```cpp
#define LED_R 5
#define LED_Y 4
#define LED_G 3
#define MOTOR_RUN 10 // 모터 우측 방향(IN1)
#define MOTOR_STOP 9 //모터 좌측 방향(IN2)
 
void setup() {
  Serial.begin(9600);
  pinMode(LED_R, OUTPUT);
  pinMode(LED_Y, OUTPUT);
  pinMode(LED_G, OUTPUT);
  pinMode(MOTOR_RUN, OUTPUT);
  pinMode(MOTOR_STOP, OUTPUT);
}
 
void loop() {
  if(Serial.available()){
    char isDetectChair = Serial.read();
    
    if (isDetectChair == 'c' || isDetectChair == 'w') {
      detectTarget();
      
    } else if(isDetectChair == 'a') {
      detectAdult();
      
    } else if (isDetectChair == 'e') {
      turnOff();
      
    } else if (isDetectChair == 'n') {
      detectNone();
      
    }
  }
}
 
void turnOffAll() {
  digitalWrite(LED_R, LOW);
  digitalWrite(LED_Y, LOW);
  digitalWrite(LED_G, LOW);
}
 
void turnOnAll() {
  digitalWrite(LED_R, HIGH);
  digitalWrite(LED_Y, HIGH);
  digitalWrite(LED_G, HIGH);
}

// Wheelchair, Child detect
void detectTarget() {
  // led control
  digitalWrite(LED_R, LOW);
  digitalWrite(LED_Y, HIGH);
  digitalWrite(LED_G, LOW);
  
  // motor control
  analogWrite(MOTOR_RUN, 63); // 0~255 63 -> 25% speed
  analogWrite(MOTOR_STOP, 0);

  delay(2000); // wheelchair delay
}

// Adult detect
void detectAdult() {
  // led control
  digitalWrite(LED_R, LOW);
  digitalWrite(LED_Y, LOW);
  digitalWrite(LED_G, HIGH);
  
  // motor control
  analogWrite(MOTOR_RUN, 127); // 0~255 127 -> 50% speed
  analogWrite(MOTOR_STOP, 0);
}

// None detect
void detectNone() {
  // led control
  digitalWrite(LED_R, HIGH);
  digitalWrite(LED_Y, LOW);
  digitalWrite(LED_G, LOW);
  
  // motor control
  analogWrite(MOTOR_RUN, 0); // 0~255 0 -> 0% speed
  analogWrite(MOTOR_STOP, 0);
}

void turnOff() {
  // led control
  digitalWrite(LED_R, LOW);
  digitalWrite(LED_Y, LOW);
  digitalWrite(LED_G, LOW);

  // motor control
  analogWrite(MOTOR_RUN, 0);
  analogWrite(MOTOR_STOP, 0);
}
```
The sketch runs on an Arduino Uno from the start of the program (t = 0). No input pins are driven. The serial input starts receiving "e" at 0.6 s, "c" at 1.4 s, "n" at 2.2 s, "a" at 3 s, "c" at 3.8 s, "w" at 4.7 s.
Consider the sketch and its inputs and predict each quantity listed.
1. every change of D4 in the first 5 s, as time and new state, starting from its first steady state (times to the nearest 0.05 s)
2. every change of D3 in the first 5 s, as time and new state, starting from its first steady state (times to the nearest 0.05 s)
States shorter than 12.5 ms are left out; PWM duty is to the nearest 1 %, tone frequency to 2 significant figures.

0 s low; 1.4 s high; 3.4 s low; 3.8 s high
0 s low; 3.4 s high; 3.8 s low
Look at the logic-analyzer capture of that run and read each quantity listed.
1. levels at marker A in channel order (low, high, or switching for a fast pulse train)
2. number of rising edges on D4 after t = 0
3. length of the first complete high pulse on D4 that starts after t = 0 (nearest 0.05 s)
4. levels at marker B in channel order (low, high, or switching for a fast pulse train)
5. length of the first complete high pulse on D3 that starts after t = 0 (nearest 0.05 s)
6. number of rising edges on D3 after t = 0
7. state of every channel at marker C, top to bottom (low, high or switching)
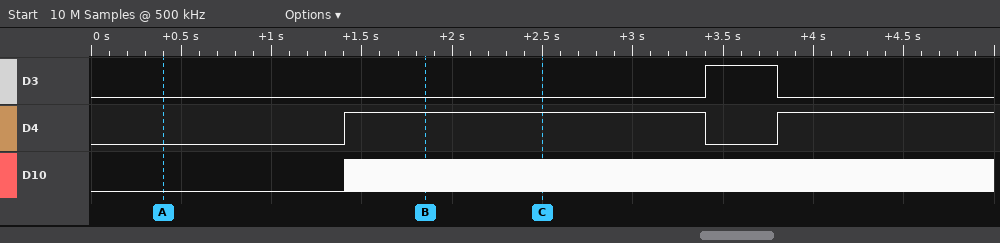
D3 low, D4 low, D10 low
2
2.00 s
D3 low, D4 high, D10 switching
0.40 s
1
D3 low, D4 high, D10 switching
